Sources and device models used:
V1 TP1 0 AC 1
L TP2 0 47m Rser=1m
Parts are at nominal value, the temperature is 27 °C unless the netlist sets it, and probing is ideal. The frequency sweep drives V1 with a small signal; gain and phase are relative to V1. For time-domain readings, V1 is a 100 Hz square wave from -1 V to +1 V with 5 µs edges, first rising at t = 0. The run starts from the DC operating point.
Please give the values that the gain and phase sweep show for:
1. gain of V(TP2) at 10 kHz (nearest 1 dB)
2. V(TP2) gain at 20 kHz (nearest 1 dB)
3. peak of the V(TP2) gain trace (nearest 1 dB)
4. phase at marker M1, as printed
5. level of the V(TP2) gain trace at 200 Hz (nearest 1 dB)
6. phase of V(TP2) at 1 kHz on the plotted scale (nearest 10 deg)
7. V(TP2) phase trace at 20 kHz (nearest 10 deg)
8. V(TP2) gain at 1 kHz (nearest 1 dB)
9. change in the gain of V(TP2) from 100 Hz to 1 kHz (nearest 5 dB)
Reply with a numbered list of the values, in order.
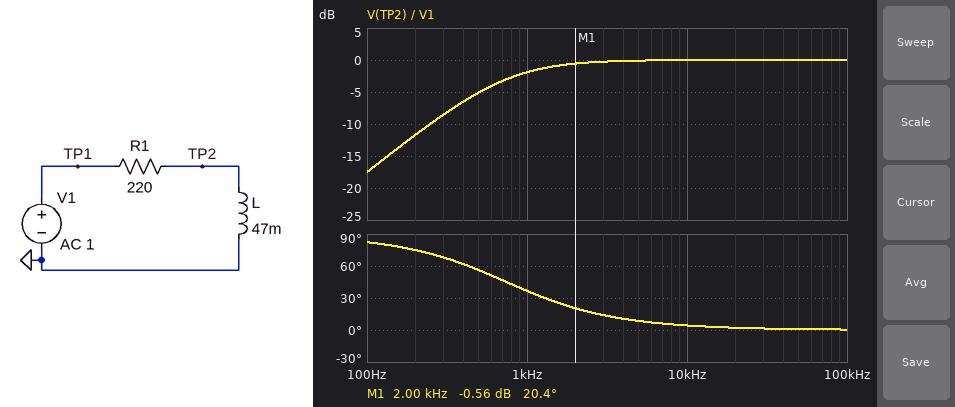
1. 0 dB
2. 0 dB
3. 0 dB
4. 20.4 deg
5. -12 dB
6. 40 deg
7. 0 deg
8. -2 dB
9. 15 dB
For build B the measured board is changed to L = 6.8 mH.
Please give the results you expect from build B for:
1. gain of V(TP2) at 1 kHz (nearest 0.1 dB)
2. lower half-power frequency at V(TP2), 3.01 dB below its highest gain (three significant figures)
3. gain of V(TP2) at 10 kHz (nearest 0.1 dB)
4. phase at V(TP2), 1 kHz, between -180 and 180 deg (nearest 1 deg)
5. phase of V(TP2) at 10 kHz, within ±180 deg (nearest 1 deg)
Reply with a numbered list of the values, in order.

1. -14.4 dB
2. 5.15 kHz
3. -1.0 dB
4. 79 deg
5. 27 deg
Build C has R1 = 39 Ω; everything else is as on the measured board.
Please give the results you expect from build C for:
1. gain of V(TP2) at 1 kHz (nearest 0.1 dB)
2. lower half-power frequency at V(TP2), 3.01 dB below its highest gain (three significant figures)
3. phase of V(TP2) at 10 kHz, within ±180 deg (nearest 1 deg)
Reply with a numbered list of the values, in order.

1. -0.1 dB
2. 132 Hz
3. 1 deg
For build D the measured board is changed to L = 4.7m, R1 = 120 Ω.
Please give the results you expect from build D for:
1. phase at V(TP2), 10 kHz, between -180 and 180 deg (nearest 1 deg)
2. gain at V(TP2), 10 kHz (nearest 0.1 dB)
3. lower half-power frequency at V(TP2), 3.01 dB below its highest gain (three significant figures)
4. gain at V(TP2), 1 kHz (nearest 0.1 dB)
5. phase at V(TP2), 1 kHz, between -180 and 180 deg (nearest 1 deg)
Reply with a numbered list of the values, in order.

1. 22 deg
2. -0.7 dB
3. 4.06 kHz
4. -12.4 dB
5. 76 deg
